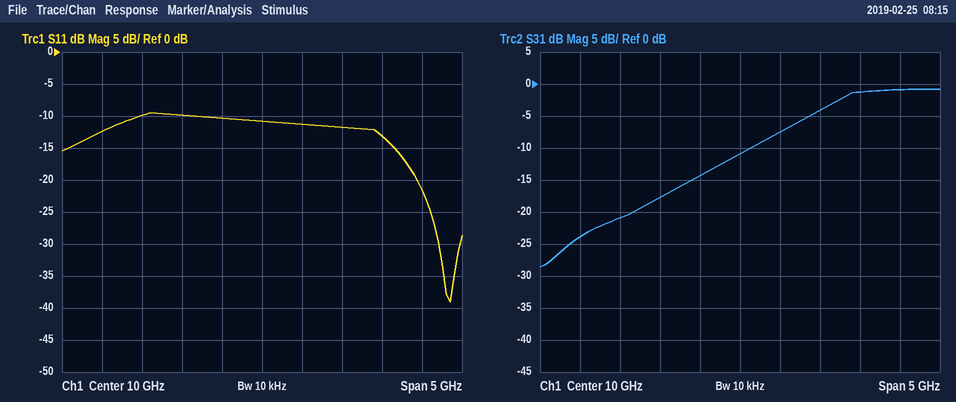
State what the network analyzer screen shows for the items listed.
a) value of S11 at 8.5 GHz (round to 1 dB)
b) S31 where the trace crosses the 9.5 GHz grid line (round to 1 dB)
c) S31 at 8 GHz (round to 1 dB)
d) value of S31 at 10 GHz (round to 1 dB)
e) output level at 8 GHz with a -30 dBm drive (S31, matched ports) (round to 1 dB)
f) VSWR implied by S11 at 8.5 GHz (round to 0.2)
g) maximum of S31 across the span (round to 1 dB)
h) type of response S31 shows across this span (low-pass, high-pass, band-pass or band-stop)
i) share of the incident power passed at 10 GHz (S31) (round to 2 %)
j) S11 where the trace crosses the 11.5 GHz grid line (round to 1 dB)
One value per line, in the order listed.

-10 dB
-14 dB
-24 dB
-11 dB
-54 dBm
2.0
-1 dB
high-pass
8 %
-13 dB
